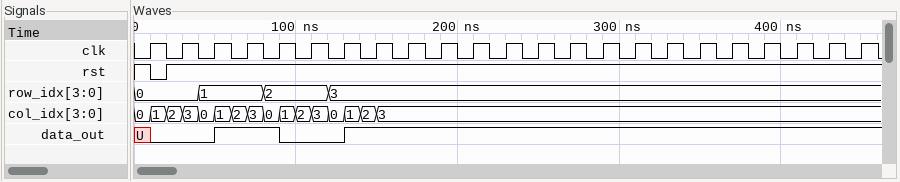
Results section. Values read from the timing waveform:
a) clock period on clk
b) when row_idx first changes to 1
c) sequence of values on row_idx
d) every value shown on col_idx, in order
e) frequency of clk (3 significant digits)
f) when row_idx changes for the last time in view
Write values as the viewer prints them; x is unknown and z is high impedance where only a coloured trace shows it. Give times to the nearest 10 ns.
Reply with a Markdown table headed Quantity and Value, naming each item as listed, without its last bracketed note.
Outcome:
| Quantity | Value |
|---|---|
| clock period on clk | 20 ns |
| when row_idx first changes to 1 | 40 ns |
| sequence of values on row_idx | 0, 1, 2, 3 |
| every value shown on col_idx, in order | 0, 1, 2, 3, 0, 1, 2, 3, 0, 1, 2, 3, 0, 1, 2, 3 |
| frequency of clk | 50.0 MHz |
| when row_idx changes for the last time in view | 120 ns |
